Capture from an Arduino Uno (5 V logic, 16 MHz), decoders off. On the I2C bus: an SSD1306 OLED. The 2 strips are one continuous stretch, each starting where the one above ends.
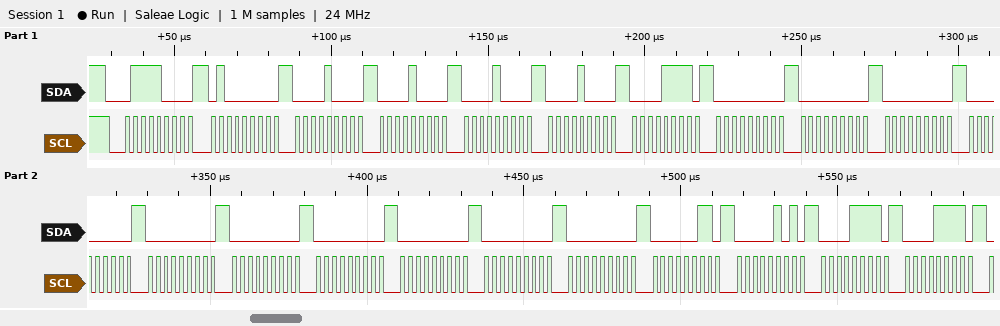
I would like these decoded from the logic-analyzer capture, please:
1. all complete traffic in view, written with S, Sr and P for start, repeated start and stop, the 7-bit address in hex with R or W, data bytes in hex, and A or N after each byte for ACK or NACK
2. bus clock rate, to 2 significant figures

S 3CW A 40 A 08 A 08 A 08 A 08 A 0F A 00 A 00 A 00 A 00 A 00 A 00 A 00 A 00 A 00 A 00 A 03 A 05 A 0F A 0F A
400 kHz
